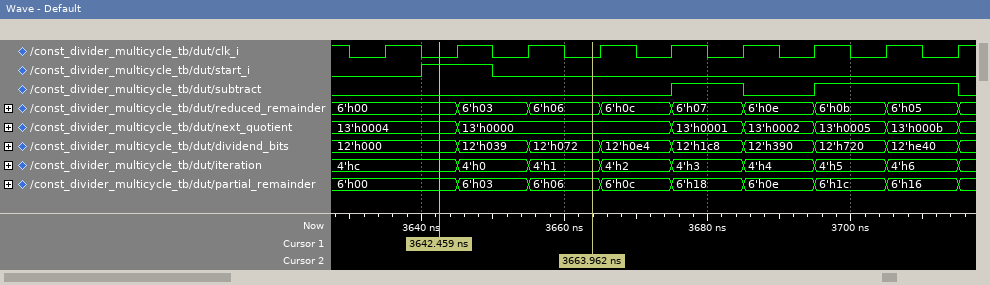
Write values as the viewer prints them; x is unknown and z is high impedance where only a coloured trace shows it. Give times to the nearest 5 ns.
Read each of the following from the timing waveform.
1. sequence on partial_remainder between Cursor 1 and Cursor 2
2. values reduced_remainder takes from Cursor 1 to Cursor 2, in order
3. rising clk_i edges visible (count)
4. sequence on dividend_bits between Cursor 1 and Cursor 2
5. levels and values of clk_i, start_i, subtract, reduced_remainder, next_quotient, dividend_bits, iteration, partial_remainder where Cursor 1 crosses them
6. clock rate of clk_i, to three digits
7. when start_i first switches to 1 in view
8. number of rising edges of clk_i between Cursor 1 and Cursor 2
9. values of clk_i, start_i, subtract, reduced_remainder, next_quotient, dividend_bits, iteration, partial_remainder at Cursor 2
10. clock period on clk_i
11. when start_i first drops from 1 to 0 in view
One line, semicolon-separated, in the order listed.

6'h00, 6'h03, 6'h06; 6'h00, 6'h03, 6'h06; 9; 12'h000, 12'h039, 12'h072; clk_i=0, start_i=1, subtract=0, reduced_remainder=6'h00, next_quotient=13'h0004, dividend_bits=12'h000, iteration=4'hc, partial_remainder=6'h00; 100 MHz; 3640 ns; 2; clk_i=0, start_i=0, subtract=0, reduced_remainder=6'h06, next_quotient=13'h0000, dividend_bits=12'h072, iteration=4'h1, partial_remainder=6'h06; 10 ns; 3650 ns
